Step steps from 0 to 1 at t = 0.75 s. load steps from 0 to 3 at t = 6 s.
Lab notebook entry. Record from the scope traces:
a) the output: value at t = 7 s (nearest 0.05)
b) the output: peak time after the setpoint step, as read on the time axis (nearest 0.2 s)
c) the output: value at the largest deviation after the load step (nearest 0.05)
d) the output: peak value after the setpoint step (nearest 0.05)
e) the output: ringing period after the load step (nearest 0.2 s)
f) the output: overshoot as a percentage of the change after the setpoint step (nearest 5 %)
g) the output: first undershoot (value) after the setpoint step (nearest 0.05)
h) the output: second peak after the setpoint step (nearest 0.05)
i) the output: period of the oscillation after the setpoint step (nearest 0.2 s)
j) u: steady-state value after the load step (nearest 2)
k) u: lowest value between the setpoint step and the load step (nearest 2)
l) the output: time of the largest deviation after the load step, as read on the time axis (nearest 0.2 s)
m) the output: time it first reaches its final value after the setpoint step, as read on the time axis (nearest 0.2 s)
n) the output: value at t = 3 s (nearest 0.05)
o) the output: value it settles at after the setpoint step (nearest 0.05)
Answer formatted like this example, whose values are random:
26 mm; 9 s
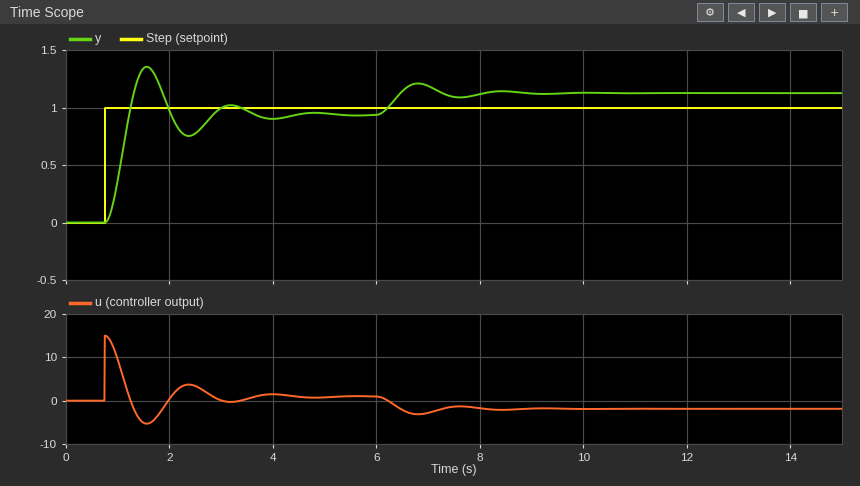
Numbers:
1.20; 1.6 s; 1.20; 1.35; 1.6 s; 45 %; 0.75; 1.00; 1.6 s; -2; -6; 6.8 s; 1.2 s; 1.00; 0.95
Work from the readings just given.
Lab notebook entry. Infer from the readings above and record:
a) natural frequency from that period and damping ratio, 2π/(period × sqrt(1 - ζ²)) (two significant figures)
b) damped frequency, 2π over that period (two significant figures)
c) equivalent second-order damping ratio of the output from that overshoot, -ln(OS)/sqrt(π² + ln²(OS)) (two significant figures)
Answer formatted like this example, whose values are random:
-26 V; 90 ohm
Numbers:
4.1 rad/s; 3.9 rad/s; 0.25
